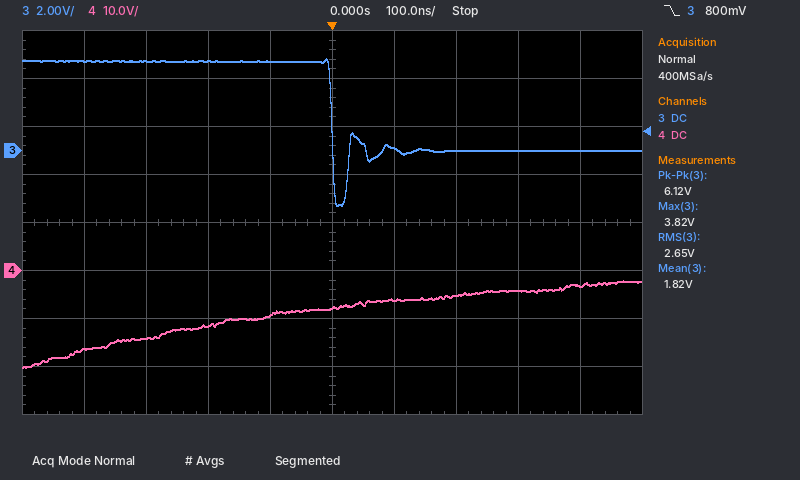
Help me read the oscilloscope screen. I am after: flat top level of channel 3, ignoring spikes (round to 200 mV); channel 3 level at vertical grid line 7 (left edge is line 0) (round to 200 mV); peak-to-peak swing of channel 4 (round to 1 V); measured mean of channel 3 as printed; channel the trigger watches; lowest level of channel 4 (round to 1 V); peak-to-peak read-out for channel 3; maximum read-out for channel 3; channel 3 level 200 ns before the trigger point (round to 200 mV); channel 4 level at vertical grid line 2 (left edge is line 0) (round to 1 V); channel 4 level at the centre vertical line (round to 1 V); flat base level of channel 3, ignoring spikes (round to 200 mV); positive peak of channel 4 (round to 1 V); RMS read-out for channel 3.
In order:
3.8 V
0.0 V
18 V
1.82 V
channel 3
-20 V
6.12 V
3.82 V
3.8 V
-14 V
-8 V
0.0 V
-2 V
2.65 V
